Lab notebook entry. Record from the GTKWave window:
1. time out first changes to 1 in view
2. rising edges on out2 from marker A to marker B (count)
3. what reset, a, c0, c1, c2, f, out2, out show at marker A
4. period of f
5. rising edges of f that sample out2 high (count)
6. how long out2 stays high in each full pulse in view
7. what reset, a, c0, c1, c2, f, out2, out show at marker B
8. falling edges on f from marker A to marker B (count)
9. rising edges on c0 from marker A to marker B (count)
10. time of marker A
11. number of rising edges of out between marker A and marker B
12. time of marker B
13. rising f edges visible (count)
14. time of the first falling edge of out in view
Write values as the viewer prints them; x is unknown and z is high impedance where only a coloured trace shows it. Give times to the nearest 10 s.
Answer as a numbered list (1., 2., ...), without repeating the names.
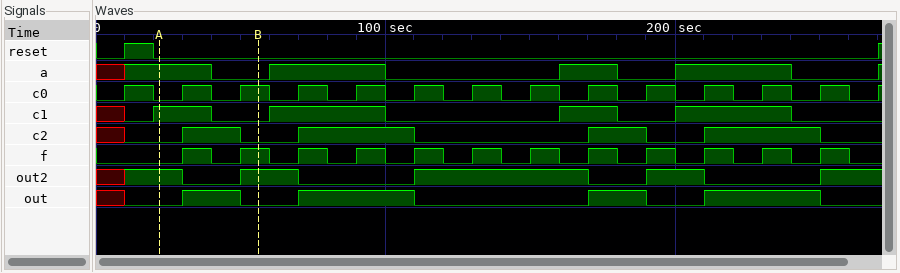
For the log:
1. 30 s
2. 1
3. reset=0, a=1, c0=0, c1=1, c2=0, f=0, out2=1, out=0
4. 20 s
5. 6
6. 20 s, 60 s, 20 s
7. reset=0, a=0, c0=1, c1=0, c2=0, f=1, out2=1, out=0
8. 1
9. 2
10. 20 s
11. 1
12. 60 s
13. 12
14. 50 s
